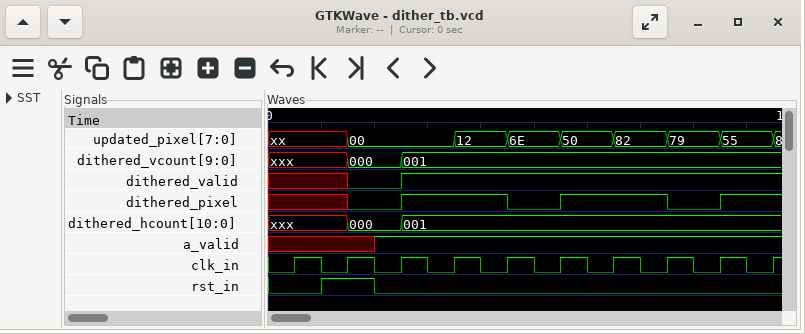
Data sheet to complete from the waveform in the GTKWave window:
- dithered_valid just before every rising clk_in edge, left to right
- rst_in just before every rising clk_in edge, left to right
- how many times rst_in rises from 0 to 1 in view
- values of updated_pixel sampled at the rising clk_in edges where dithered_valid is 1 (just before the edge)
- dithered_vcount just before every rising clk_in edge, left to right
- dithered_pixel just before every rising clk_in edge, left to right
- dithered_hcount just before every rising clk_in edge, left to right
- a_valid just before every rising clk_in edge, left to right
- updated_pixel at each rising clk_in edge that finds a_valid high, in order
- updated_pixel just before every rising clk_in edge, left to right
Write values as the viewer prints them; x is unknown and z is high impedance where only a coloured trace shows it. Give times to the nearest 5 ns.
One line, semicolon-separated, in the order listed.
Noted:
x x 0 1 1 1 1 1 1 1; 0 1 0 0 0 0 0 0 0 0; 1; 00, 12, 6E, 50, 82, 79, 55; xxx, xxx, 000, 001, 001, 001, 001, 001, 001, 001; x x 0 1 1 0 1 1 0 1; xxx, xxx, 000, 001, 001, 001, 001, 001, 001, 001; x x 1 1 1 1 1 1 1 1; 00, 00, 12, 6E, 50, 82, 79, 55; xx, xx, 00, 00, 12, 6E, 50, 82, 79, 55
